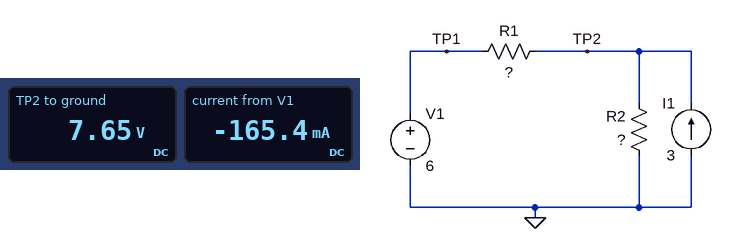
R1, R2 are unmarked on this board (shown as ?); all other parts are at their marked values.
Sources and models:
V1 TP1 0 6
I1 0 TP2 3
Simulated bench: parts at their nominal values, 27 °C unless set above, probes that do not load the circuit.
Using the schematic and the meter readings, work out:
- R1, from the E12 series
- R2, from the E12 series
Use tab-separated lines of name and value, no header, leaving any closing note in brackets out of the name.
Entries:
R1, from the E12 series	10 Ω
R2, from the E12 series	2.7 Ω
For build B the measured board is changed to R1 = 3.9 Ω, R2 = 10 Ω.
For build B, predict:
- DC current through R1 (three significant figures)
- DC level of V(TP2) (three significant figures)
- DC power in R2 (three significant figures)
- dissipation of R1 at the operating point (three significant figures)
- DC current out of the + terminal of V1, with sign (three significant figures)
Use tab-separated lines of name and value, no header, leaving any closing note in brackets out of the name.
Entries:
DC current through R1	1.73 A
DC level of V(TP2)	12.7 V
DC power in R2	16.2 W
dissipation of R1 at the operating point	11.6 W
DC current out of the + terminal of V1, with sign	-1.73 A
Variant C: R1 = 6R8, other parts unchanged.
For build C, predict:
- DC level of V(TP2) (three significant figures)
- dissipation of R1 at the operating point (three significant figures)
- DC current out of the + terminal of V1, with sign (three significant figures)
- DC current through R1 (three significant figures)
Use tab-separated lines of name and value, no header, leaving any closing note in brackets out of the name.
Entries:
DC level of V(TP2)	7.50 V
dissipation of R1 at the operating point	332 mW
DC current out of the + terminal of V1, with sign	-221 mA
DC current through R1	221 mA
